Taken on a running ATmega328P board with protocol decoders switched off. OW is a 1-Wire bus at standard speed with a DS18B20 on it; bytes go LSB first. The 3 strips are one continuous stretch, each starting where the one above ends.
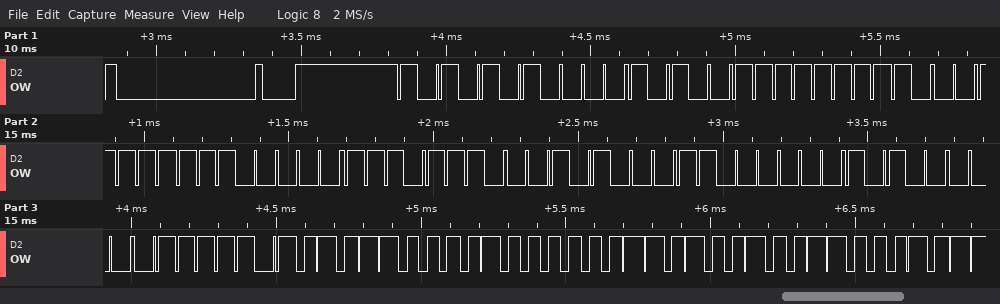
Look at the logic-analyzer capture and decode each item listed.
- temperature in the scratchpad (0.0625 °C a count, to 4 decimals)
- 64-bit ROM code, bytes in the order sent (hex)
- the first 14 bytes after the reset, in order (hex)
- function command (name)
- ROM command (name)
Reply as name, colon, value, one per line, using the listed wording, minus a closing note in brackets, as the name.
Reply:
temperature in the scratchpad: 33.6250 °C
64-bit ROM code, bytes in the order sent: 28 FF F1 07 77 14 03 05
the first 14 bytes after the reset, in order: 55 28 FF F1 07 77 14 03 05 BE 1A 02 4B 46
function command: Read Scratchpad
ROM command: Match ROM
